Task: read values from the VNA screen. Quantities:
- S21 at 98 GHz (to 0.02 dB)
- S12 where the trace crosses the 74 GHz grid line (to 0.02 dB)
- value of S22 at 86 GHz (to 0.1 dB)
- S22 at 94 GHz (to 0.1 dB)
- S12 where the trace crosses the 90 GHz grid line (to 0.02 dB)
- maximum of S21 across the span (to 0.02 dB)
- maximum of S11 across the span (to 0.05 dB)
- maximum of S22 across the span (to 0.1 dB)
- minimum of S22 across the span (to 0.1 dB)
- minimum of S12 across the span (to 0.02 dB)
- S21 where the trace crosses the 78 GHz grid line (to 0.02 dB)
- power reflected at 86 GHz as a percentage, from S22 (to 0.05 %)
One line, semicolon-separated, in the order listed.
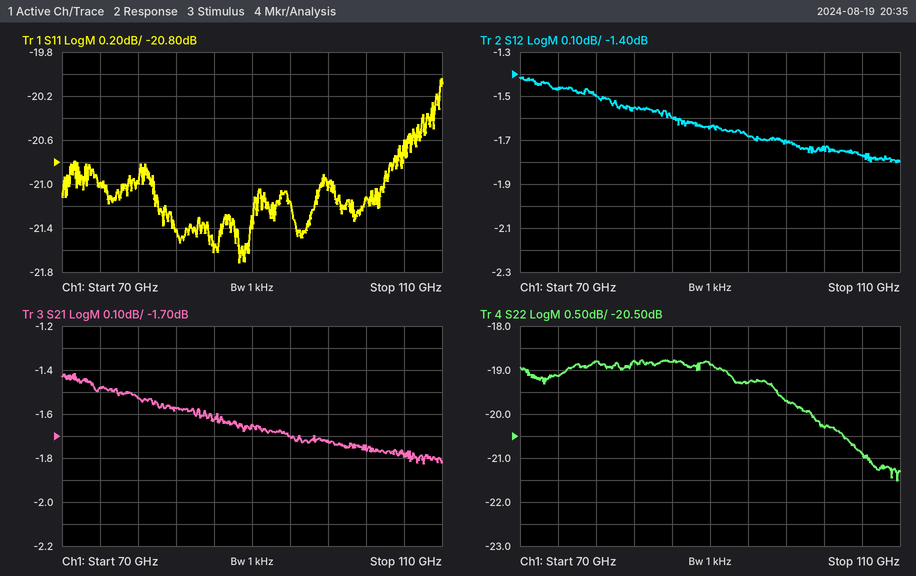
-1.72 dB; -1.46 dB; -18.8 dB; -19.3 dB; -1.64 dB; -1.42 dB; -20.05 dB; -18.8 dB; -21.5 dB; -1.80 dB; -1.52 dB; 1.30 %
